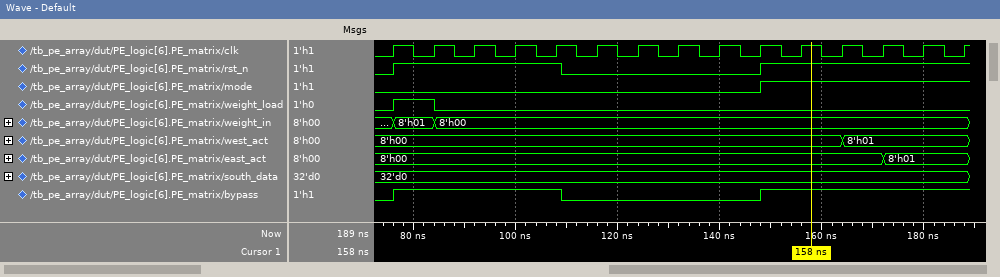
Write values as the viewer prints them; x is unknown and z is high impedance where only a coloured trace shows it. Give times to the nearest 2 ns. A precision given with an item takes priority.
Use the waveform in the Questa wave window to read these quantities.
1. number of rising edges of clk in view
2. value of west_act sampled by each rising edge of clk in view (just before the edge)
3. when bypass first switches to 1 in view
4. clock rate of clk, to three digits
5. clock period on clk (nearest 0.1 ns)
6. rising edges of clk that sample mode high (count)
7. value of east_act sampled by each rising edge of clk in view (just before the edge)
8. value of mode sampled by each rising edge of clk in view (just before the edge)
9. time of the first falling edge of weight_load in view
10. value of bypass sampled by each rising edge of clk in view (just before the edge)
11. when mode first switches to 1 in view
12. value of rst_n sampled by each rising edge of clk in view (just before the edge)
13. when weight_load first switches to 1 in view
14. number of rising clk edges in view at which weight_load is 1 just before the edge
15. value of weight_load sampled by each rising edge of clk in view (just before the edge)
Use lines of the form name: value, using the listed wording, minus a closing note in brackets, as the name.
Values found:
number of rising edges of clk in view: 15
value of west_act sampled by each rising edge of clk in view: 8'h00, 8'h00, 8'h00, 8'h00, 8'h00, 8'h00, 8'h00, 8'h00, 8'h00, 8'h00, 8'h00, 8'h00, 8'h01, 8'h01, 8'h01
when bypass first switches to 1 in view: 76 ns
clock rate of clk, to three digits: 125 MHz
clock period on clk: 8 ns
rising edges of clk that sample mode high: 5
value of east_act sampled by each rising edge of clk in view: 8'h00, 8'h00, 8'h00, 8'h00, 8'h00, 8'h00, 8'h00, 8'h00, 8'h00, 8'h00, 8'h00, 8'h00, 8'h00, 8'h01, 8'h01
value of mode sampled by each rising edge of clk in view: 0 0 0 0 0 0 0 0 0 0 1 1 1 1 1
time of the first falling edge of weight_load in view: 84 ns
value of bypass sampled by each rising edge of clk in view: 0 1 1 1 1 0 0 0 0 0 1 1 1 1 1
when mode first switches to 1 in view: 148 ns
value of rst_n sampled by each rising edge of clk in view: 0 1 1 1 1 0 0 0 0 0 1 1 1 1 1
when weight_load first switches to 1 in view: 76 ns
number of rising clk edges in view at which weight_load is 1 just before the edge: 1
value of weight_load sampled by each rising edge of clk in view: 0 1 0 0 0 0 0 0 0 0 0 0 0 0 0
